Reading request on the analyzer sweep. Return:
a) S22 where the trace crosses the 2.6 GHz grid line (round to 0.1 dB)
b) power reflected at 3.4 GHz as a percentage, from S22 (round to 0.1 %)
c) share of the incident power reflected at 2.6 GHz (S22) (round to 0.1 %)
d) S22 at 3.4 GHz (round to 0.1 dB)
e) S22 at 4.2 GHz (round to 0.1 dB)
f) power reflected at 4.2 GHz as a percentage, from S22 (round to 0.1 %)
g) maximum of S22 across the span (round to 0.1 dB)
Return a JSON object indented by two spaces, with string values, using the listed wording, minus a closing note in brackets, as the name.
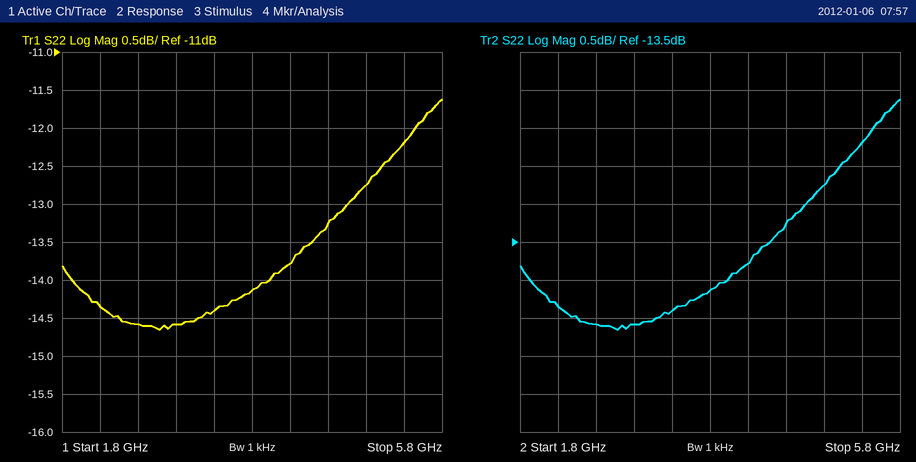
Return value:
{
  "S22 where the trace crosses the 2.6 GHz grid line": "-14.6 dB",
  "power reflected at 3.4 GHz as a percentage, from S22": "3.6 %",
  "share of the incident power reflected at 2.6 GHz (S22)": "3.5 %",
  "S22 at 3.4 GHz": "-14.4 dB",
  "S22 at 4.2 GHz": "-13.8 dB",
  "power reflected at 4.2 GHz as a percentage, from S22": "4.2 %",
  "maximum of S22 across the span": "-11.6 dB"
}
